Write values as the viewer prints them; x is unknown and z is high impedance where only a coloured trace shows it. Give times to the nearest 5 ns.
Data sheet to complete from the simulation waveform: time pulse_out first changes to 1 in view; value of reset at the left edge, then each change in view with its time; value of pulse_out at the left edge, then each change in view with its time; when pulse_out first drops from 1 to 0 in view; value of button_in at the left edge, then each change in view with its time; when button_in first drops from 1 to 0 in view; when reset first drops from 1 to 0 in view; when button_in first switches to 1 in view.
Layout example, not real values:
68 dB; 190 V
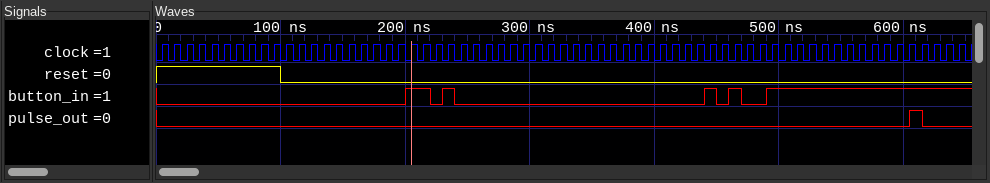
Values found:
605 ns; 1, 0 at 100 ns; 0, 1 at 605 ns, 0 at 615 ns; 615 ns; 0, 1 at 200 ns, 0 at 220 ns, 1 at 230 ns, 0 at 240 ns, 1 at 440 ns, 0 at 450 ns, 1 at 460 ns, 0 at 470 ns, 1 at 490 ns; 220 ns; 100 ns; 200 ns
